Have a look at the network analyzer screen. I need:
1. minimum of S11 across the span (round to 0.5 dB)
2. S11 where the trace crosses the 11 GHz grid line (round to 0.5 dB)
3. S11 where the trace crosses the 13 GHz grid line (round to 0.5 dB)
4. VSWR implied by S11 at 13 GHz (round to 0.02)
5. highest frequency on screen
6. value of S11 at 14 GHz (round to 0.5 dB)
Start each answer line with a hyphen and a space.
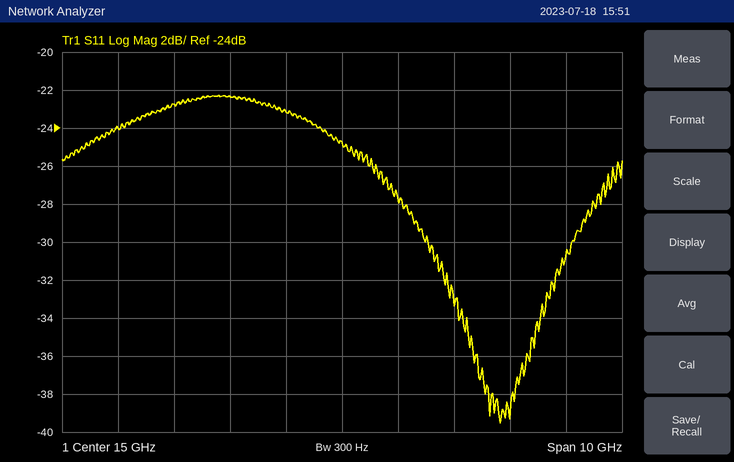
- -39.5 dB
- -24.0 dB
- -22.5 dB
- 1.16
- 20 GHz
- -23.0 dB
